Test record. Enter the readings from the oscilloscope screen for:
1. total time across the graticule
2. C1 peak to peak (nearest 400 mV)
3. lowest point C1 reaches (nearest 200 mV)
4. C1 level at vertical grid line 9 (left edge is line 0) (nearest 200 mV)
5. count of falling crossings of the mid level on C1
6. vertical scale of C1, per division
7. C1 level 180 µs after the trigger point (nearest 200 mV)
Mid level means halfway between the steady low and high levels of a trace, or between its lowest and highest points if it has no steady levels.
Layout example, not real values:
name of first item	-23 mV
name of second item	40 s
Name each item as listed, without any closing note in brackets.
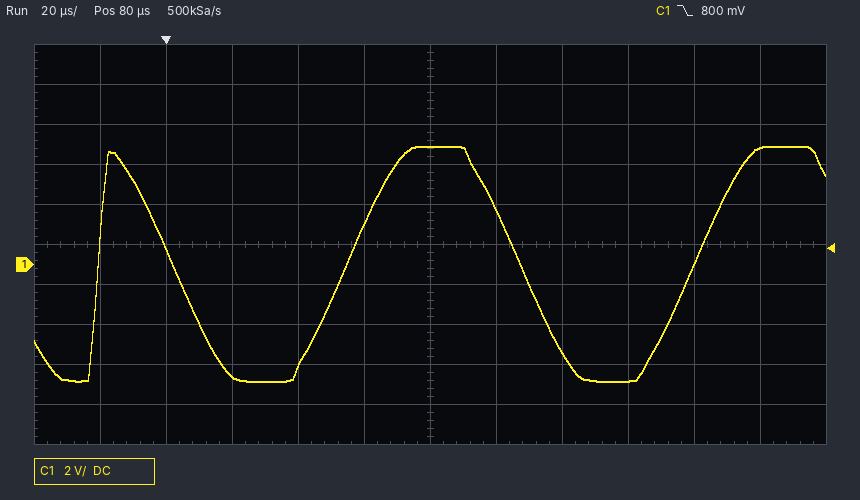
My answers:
total time across the graticule	240 µs
C1 peak to peak	11.6 V
lowest point C1 reaches	-5.8 V
C1 level at vertical grid line 9 (left edge is line 0)	-5.8 V
count of falling crossings of the mid level on C1	2
vertical scale of C1, per division	2 V
C1 level 180 µs after the trigger point	5.8 V
